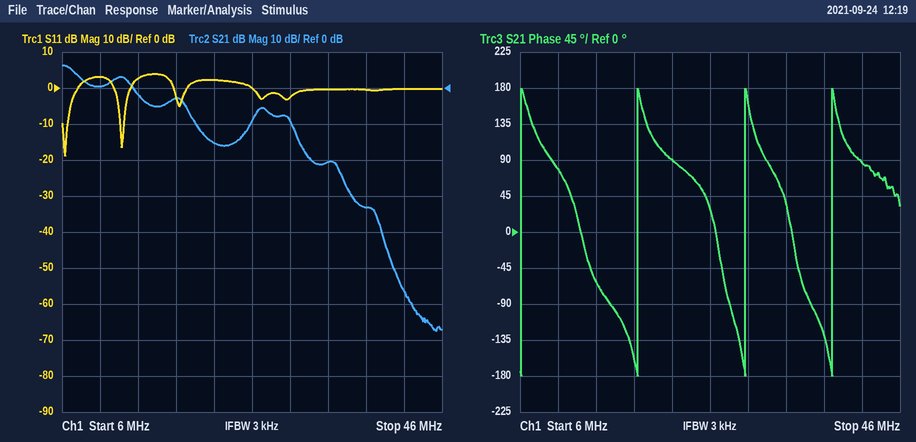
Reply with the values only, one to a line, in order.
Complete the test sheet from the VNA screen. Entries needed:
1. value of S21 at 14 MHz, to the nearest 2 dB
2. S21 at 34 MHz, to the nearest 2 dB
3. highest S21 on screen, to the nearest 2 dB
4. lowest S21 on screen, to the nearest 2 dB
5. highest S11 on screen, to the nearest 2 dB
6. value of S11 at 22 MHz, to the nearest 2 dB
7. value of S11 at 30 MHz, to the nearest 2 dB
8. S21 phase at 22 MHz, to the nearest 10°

-2 dB
-20 dB
6 dB
-68 dB
4 dB
2 dB
-2 dB
90°
